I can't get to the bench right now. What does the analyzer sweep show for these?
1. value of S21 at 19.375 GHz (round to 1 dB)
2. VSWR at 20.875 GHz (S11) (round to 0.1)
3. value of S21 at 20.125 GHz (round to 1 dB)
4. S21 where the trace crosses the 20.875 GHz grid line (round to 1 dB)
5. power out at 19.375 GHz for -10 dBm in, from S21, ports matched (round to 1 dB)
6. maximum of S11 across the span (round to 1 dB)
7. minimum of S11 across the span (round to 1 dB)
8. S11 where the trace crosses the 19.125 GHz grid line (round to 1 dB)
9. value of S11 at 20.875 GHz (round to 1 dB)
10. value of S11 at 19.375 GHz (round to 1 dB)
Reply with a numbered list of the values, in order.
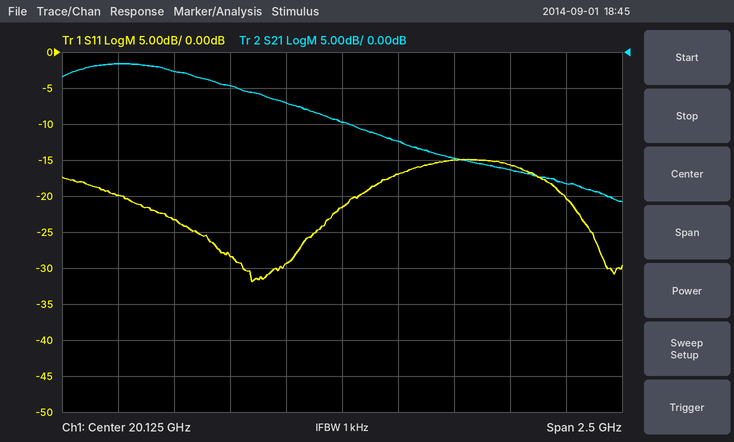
1. -3 dB
2. 1.4
3. -10 dB
4. -16 dB
5. -13 dBm
6. -15 dB
7. -32 dB
8. -20 dB
9. -16 dB
10. -23 dB
